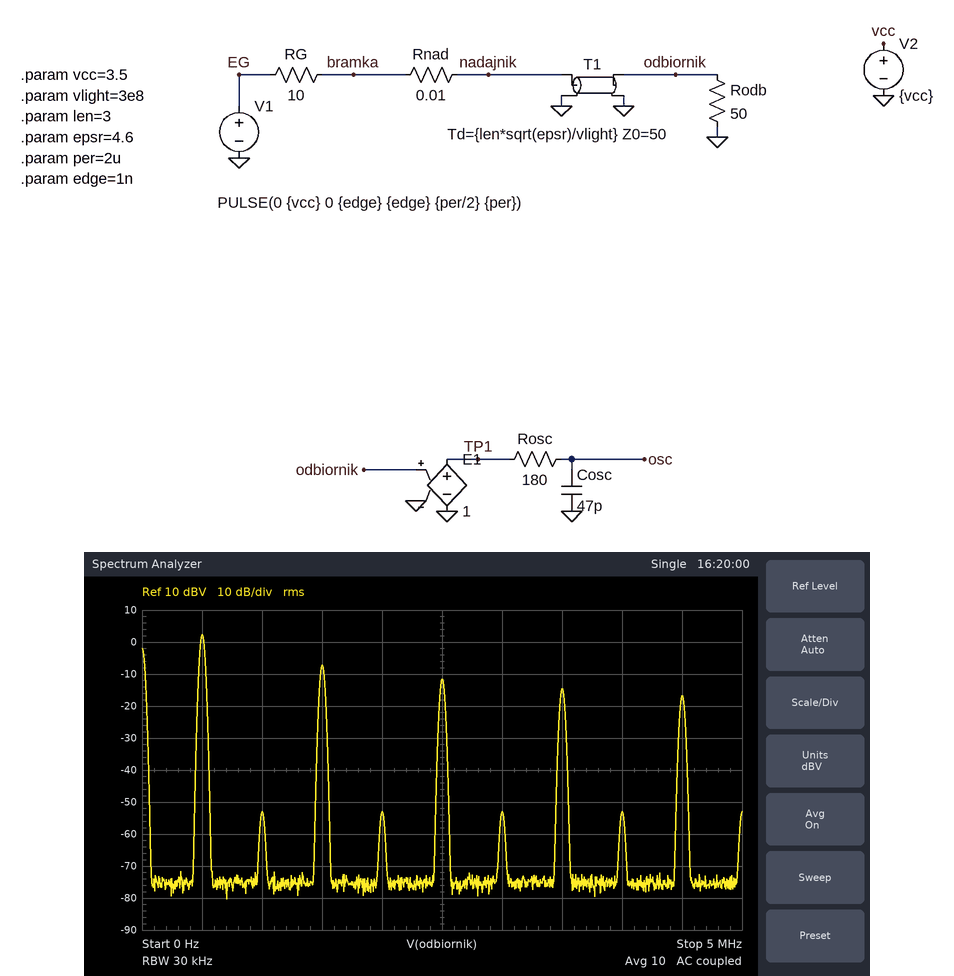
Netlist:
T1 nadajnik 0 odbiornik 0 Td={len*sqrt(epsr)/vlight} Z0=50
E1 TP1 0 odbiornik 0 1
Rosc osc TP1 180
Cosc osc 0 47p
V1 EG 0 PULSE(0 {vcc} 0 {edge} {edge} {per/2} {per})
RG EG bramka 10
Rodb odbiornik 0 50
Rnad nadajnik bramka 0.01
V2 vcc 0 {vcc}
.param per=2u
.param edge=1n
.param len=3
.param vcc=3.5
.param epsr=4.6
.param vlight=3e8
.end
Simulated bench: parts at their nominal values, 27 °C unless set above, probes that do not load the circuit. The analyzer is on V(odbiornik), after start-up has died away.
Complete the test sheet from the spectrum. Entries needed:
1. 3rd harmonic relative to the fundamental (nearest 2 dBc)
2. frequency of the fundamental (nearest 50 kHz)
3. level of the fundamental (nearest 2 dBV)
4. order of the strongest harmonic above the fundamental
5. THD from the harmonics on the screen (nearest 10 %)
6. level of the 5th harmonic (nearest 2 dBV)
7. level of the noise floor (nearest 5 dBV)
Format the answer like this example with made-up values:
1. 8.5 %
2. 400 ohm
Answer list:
1. -10 dBc
2. 500 kHz
3. 2 dBV
4. 3
5. 40 %
6. -12 dBV
7. -75 dBV
